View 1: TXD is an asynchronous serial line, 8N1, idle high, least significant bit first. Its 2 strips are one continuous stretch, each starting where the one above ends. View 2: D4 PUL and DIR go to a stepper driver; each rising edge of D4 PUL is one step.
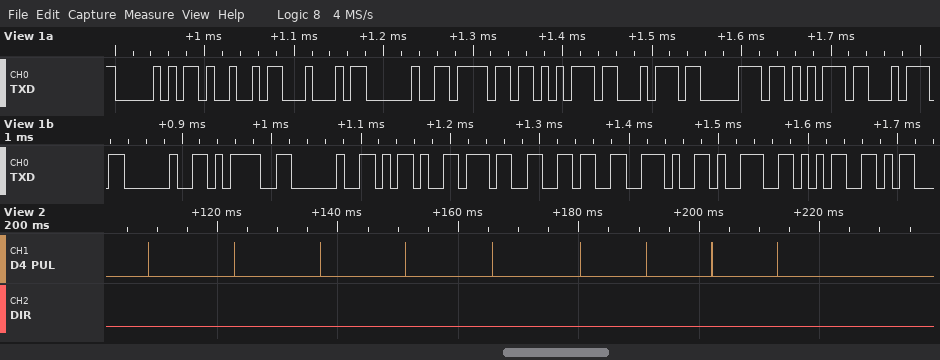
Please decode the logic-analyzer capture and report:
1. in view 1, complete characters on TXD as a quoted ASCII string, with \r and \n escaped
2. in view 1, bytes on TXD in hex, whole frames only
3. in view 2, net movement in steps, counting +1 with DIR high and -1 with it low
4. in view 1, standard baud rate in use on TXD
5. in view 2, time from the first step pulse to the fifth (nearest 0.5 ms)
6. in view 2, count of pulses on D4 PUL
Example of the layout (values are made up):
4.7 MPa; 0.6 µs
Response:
"PID output = -76.95"; 50 49 44 20 6F 75 74 70 75 74 20 3D 20 2D 37 36 2E 39 35; -9; 115200 baud; 57.0 ms; 9
